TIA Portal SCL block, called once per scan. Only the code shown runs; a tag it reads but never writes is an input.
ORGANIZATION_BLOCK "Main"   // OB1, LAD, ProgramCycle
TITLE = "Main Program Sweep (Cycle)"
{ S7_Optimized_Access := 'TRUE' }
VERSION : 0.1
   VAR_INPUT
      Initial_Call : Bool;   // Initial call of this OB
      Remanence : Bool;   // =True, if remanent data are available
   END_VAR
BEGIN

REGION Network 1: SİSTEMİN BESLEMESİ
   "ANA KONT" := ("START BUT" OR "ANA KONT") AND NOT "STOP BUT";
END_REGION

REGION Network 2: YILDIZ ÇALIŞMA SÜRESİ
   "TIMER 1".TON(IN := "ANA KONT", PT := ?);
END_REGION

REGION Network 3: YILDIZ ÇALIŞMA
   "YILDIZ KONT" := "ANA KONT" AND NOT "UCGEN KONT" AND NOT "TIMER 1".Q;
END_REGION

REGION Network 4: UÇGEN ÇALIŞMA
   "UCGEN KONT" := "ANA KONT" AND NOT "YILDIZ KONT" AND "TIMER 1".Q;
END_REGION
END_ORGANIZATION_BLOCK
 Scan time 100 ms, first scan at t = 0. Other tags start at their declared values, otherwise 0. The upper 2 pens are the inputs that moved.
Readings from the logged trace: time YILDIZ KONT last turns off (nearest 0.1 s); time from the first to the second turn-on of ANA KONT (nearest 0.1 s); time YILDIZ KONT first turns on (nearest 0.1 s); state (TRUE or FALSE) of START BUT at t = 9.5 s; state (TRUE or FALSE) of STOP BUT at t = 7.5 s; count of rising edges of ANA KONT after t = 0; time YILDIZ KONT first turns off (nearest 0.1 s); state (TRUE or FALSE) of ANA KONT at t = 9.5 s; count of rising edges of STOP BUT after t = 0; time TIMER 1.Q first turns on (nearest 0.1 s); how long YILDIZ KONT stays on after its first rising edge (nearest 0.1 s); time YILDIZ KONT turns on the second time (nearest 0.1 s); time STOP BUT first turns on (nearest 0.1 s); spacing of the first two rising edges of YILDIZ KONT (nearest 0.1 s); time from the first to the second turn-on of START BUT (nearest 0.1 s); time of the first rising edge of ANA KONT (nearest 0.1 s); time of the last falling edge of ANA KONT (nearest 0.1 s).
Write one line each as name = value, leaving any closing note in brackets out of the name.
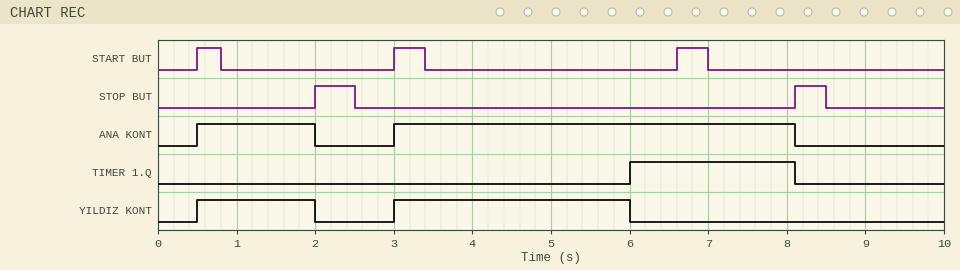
time YILDIZ KONT last turns off = 6.0 s
time from the first to the second turn-on of ANA KONT = 2.5 s
time YILDIZ KONT first turns on = 0.5 s
state (TRUE or FALSE) of START BUT at t = 9.5 s = FALSE
state (TRUE or FALSE) of STOP BUT at t = 7.5 s = FALSE
count of rising edges of ANA KONT after t = 0 = 2
time YILDIZ KONT first turns off = 2.0 s
state (TRUE or FALSE) of ANA KONT at t = 9.5 s = FALSE
count of rising edges of STOP BUT after t = 0 = 2
time TIMER 1.Q first turns on = 6.0 s
how long YILDIZ KONT stays on after its first rising edge = 1.5 s
time YILDIZ KONT turns on the second time = 3.0 s
time STOP BUT first turns on = 2.0 s
spacing of the first two rising edges of YILDIZ KONT = 2.5 s
time from the first to the second turn-on of START BUT = 2.5 s
time of the first rising edge of ANA KONT = 0.5 s
time of the last falling edge of ANA KONT = 8.1 s
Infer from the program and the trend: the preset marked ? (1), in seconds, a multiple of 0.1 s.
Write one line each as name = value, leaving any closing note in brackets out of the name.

the preset marked ? (1), in seconds, a multiple of 0.1 s = 3.0 s
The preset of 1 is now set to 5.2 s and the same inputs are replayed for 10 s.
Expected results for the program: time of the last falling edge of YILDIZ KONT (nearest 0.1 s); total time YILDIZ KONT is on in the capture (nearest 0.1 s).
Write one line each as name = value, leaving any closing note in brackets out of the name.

time of the last falling edge of YILDIZ KONT = 8.1 s
total time YILDIZ KONT is on in the capture = 6.6 s
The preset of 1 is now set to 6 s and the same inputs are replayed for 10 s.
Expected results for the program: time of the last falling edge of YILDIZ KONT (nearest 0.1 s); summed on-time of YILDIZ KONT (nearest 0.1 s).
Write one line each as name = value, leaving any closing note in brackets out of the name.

time of the last falling edge of YILDIZ KONT = 8.1 s
summed on-time of YILDIZ KONT = 6.6 s
